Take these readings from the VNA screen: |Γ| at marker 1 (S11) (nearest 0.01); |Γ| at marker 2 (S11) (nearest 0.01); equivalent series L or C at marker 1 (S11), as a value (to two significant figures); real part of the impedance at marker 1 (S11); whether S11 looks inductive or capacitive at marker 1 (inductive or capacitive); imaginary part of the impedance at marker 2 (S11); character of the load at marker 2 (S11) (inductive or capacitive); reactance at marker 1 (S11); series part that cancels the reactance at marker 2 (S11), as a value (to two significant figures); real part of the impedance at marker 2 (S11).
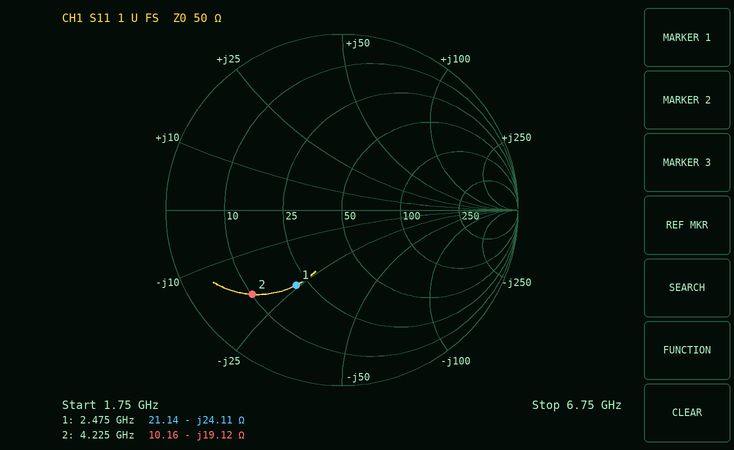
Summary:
0.50
0.70
2.7 pF
21.14 Ω
capacitive
-19.12 Ω
capacitive
-24.11 Ω
720 pH
10.16 Ω
